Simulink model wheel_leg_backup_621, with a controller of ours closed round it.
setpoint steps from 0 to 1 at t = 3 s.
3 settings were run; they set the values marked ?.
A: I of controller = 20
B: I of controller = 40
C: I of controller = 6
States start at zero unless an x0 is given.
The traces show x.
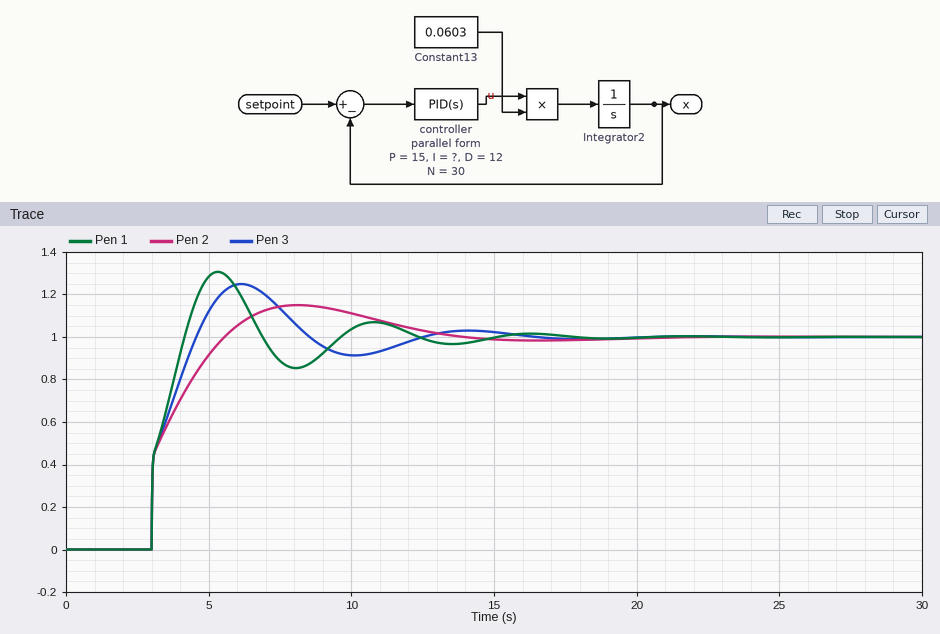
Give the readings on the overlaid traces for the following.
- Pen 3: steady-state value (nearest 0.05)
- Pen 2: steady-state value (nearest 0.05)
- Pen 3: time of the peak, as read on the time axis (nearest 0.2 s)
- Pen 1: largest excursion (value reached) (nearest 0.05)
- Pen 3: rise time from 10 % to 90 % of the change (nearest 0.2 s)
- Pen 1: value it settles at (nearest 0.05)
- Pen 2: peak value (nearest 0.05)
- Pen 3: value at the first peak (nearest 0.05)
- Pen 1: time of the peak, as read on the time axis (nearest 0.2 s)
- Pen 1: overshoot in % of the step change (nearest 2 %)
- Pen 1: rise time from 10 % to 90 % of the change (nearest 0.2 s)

1.00
1.00
6.2 s
1.30
1.2 s
1.00
1.15
1.25
5.4 s
30 %
1.0 s
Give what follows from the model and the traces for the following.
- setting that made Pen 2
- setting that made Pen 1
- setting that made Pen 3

C
B
A
